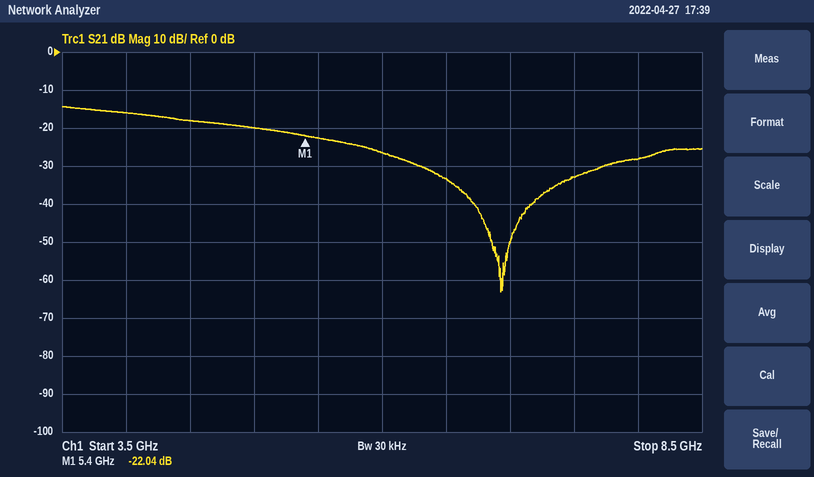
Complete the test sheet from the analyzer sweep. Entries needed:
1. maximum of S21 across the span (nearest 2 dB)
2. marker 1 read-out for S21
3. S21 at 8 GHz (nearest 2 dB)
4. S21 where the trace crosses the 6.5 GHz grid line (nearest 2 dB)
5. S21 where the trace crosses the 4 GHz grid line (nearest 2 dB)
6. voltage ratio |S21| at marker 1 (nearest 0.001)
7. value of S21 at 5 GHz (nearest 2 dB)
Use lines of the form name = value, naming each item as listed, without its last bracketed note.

maximum of S21 across the span = -14 dB
marker 1 read-out for S21 = -22.04 dB
S21 at 8 GHz = -28 dB
S21 where the trace crosses the 6.5 GHz grid line = -34 dB
S21 where the trace crosses the 4 GHz grid line = -16 dB
voltage ratio |S21| at marker 1 = 0.079
value of S21 at 5 GHz = -20 dB
